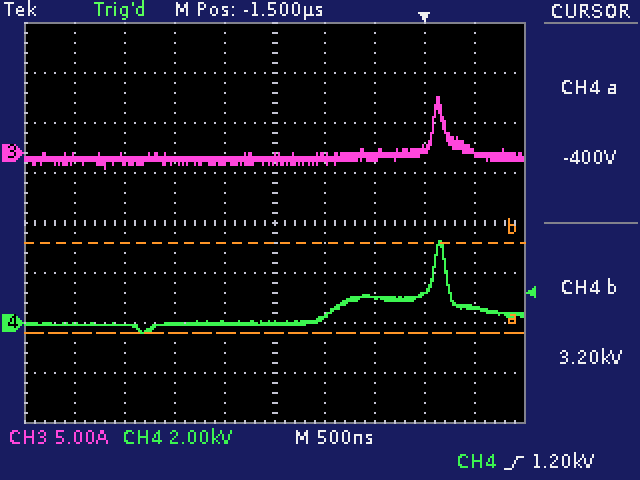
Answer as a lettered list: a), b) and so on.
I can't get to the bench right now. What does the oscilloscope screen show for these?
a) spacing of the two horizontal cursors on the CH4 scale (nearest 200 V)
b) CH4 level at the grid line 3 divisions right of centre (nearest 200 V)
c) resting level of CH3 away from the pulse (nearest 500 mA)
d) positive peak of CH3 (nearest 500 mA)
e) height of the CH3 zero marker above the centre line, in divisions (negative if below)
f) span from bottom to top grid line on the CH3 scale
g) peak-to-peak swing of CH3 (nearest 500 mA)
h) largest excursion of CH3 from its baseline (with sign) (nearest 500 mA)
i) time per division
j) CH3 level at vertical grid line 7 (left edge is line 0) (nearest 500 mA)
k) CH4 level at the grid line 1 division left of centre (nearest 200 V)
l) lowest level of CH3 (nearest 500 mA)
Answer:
a) 3.6 kV
b) 1.2 kV
c) -500 mA
d) 5.5 A
e) +1.4 div
f) 40 A
g) 7.0 A
h) +6.0 A
i) 500 ns
j) -500 mA
k) 0.0 kV
l) -1.5 A
